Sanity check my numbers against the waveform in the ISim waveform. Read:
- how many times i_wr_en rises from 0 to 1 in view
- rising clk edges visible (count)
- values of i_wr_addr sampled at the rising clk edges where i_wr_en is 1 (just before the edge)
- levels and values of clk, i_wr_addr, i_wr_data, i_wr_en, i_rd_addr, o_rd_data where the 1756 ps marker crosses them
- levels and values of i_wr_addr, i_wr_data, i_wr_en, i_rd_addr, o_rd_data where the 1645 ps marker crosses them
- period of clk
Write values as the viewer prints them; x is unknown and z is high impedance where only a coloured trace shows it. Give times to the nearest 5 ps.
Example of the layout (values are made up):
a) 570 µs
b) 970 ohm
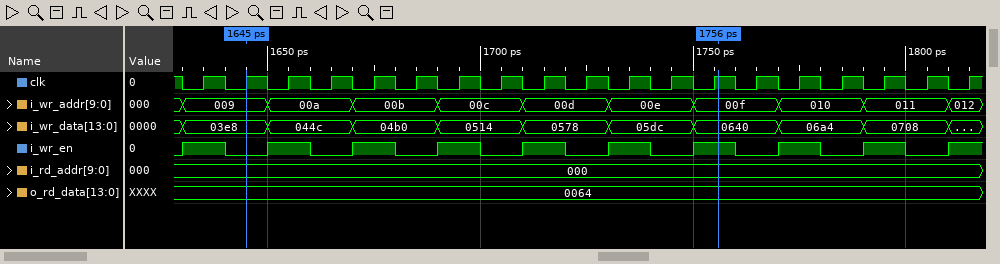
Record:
a) 10
b) 19
c) 009, 00a, 00b, 00c, 00d, 00e, 00f, 010, 011, 012
d) clk=1, i_wr_addr=00f, i_wr_data=0640, i_wr_en=1, i_rd_addr=000, o_rd_data=0064
e) i_wr_addr=009, i_wr_data=03e8, i_wr_en=0, i_rd_addr=000, o_rd_data=0064
f) 10 ps
